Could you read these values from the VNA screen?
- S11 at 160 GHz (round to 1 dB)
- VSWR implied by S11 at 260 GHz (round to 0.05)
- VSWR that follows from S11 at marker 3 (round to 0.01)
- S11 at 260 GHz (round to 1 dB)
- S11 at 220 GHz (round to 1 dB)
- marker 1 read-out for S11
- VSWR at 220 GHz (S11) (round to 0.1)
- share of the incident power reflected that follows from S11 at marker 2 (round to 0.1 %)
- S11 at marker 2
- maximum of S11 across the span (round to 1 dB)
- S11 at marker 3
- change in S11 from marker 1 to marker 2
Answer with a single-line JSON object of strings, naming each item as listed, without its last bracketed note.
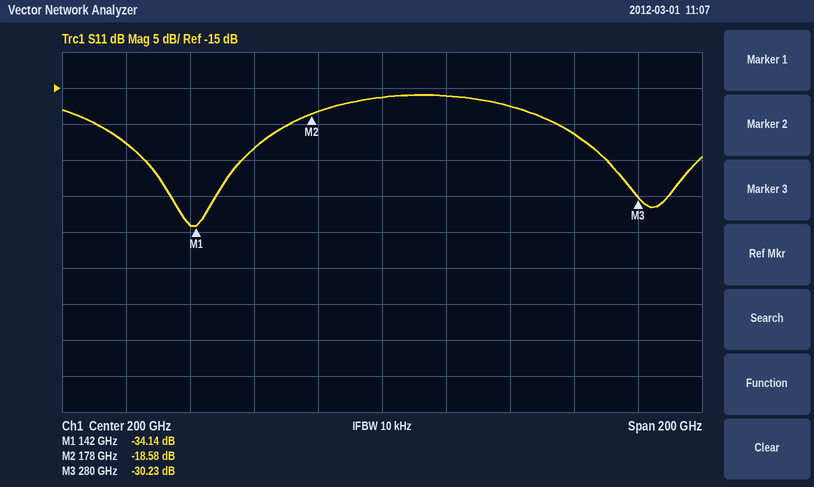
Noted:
{"S11 at 160 GHz": "-23 dB", "VSWR implied by S11 at 260 GHz": "1.20", "VSWR that follows from S11 at marker 3": "1.06", "S11 at 260 GHz": "-21 dB", "S11 at 220 GHz": "-16 dB", "marker 1 read-out for S11": "-34.14 dB", "VSWR at 220 GHz (S11)": "1.4", "share of the incident power reflected that follows from S11 at marker 2": "1.4 %", "S11 at marker 2": "-18.58 dB", "maximum of S11 across the span": "-16 dB", "S11 at marker 3": "-30.23 dB", "change in S11 from marker 1 to marker 2": "15.56 dB"}
